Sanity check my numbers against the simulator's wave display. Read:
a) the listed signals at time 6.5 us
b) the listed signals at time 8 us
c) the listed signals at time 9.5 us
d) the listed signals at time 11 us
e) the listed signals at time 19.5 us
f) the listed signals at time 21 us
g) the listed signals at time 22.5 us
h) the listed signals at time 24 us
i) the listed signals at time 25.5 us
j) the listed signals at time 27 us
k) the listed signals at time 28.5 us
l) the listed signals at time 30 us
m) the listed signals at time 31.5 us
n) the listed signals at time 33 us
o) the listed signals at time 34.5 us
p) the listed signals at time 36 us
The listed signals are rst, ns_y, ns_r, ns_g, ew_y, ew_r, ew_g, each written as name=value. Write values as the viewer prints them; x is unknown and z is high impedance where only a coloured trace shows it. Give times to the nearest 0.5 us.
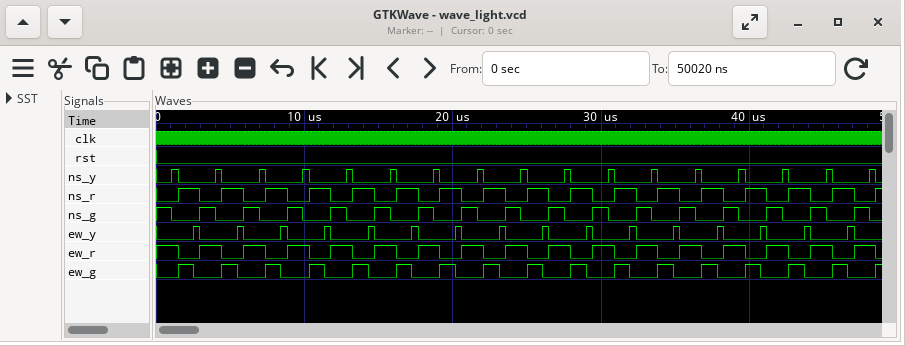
rst=0, ns_y=0, ns_r=0, ns_g=1, ew_y=0, ew_r=1, ew_g=0
rst=0, ns_y=0, ns_r=1, ns_g=0, ew_y=0, ew_r=0, ew_g=1
rst=0, ns_y=0, ns_r=0, ns_g=1, ew_y=0, ew_r=1, ew_g=0
rst=0, ns_y=0, ns_r=1, ns_g=0, ew_y=0, ew_r=0, ew_g=1
rst=0, ns_y=0, ns_r=1, ns_g=0, ew_y=0, ew_r=0, ew_g=1
rst=0, ns_y=0, ns_r=0, ns_g=1, ew_y=0, ew_r=1, ew_g=0
rst=0, ns_y=0, ns_r=1, ns_g=0, ew_y=0, ew_r=0, ew_g=1
rst=0, ns_y=0, ns_r=0, ns_g=1, ew_y=0, ew_r=1, ew_g=0
rst=0, ns_y=0, ns_r=1, ns_g=0, ew_y=0, ew_r=0, ew_g=1
rst=0, ns_y=0, ns_r=0, ns_g=1, ew_y=0, ew_r=1, ew_g=0
rst=0, ns_y=0, ns_r=1, ns_g=0, ew_y=0, ew_r=0, ew_g=1
rst=0, ns_y=0, ns_r=0, ns_g=1, ew_y=0, ew_r=1, ew_g=0
rst=0, ns_y=0, ns_r=1, ns_g=0, ew_y=0, ew_r=0, ew_g=1
rst=0, ns_y=0, ns_r=0, ns_g=1, ew_y=0, ew_r=1, ew_g=0
rst=0, ns_y=0, ns_r=1, ns_g=0, ew_y=0, ew_r=0, ew_g=1
rst=0, ns_y=0, ns_r=0, ns_g=1, ew_y=0, ew_r=1, ew_g=0
